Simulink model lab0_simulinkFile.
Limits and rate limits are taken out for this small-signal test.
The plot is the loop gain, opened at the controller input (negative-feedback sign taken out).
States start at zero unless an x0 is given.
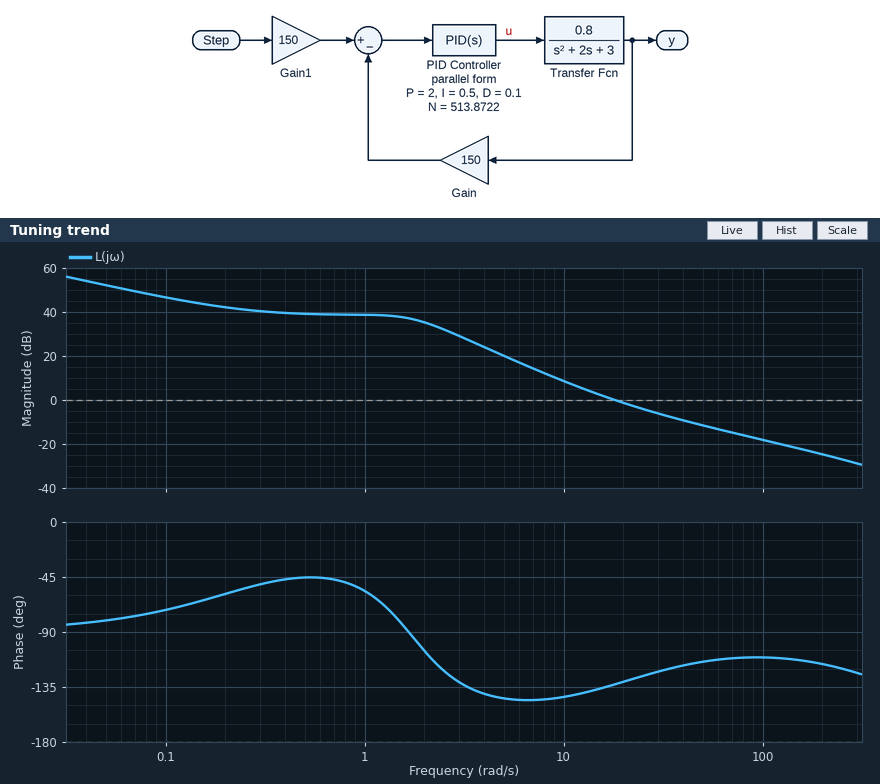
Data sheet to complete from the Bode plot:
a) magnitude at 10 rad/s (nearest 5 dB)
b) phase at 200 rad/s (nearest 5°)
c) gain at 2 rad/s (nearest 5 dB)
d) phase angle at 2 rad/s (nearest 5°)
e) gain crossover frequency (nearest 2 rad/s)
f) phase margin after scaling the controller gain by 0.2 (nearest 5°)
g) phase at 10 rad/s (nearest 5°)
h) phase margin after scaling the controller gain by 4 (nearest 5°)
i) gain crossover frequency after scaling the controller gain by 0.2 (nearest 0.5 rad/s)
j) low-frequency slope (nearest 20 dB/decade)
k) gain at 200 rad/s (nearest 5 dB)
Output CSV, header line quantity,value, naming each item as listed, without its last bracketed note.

quantity,value
magnitude at 10 rad/s,10 dB
phase at 200 rad/s,-115°
gain at 2 rad/s,35 dB
phase angle at 2 rad/s,-105°
gain crossover frequency,18 rad/s
phase margin after scaling the controller gain by 0.2,35°
phase at 10 rad/s,-145°
phase margin after scaling the controller gain by 4,65°
gain crossover frequency after scaling the controller gain by 0.2,7.0 rad/s
low-frequency slope,-20 dB/decade
gain at 200 rad/s,-25 dB
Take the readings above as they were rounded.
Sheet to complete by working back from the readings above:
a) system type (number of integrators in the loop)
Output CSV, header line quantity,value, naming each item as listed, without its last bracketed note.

quantity,value
system type,1
